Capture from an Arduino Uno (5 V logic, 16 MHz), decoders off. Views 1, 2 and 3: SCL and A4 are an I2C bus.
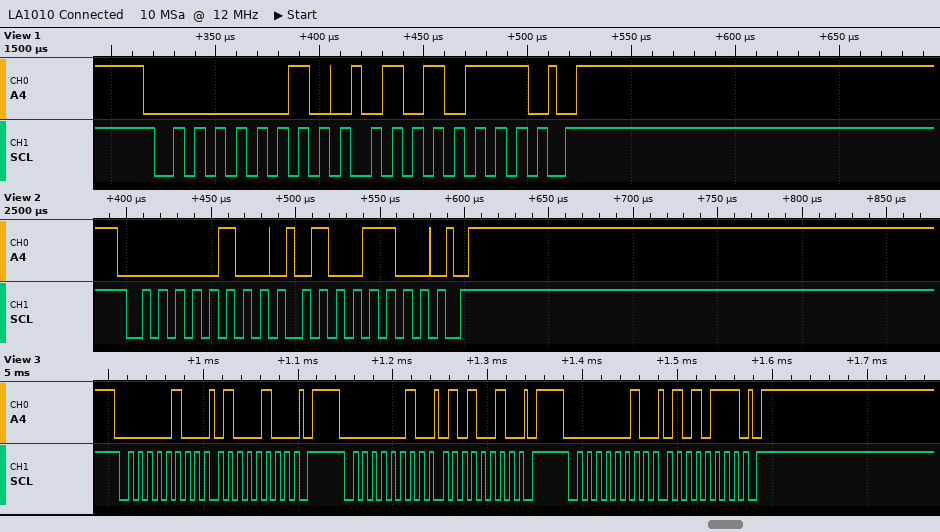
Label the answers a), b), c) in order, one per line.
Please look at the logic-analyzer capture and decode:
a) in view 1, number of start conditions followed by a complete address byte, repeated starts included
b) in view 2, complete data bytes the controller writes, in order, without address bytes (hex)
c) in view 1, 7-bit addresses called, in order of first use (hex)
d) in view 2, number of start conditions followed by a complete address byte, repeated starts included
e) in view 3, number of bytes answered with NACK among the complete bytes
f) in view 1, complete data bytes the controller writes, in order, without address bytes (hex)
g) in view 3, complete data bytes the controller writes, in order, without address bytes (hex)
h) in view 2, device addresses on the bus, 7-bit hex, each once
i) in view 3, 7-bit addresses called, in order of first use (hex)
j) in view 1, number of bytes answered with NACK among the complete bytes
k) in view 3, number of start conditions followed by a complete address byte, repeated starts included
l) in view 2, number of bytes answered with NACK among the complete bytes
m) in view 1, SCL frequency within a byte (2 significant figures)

a) 1
b) 4C
c) 0x01
d) 1
e) 0
f) 57
g) 44 52 57
h) 0x02
i) 0x02 0x01
j) 0
k) 3
l) 0
m) 100 kHz
